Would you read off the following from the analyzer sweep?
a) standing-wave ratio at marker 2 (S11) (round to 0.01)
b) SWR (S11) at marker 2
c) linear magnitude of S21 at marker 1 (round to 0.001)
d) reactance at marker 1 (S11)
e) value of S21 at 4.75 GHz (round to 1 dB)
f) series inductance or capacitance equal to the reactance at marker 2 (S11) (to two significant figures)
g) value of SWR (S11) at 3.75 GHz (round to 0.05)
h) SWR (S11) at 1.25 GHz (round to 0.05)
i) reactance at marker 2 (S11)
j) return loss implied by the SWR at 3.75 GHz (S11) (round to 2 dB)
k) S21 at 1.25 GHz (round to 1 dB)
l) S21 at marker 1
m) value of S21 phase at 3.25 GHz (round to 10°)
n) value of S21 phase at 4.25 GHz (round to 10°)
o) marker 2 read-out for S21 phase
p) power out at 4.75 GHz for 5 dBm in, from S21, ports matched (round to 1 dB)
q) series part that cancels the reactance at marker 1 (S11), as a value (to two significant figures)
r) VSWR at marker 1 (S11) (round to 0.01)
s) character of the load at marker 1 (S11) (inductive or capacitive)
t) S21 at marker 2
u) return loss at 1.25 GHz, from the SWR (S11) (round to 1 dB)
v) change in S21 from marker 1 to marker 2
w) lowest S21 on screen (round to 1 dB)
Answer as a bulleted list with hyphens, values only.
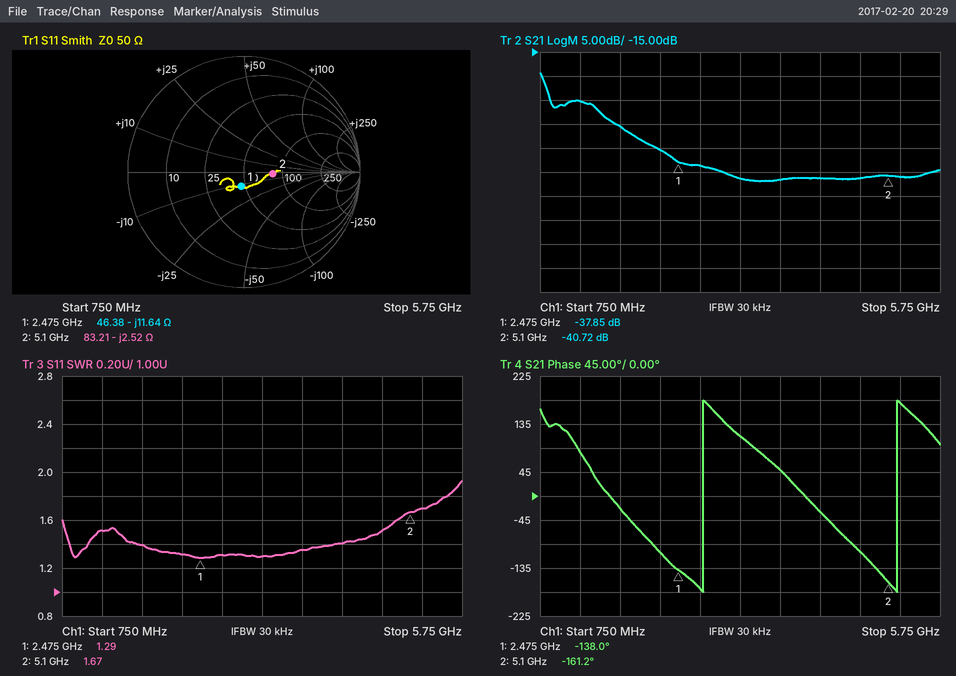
- 1.67
- 1.67
- 0.013
- -11.64 Ω
- -41 dB
- 12 pF
- 1.35
- 1.50
- -2.52 Ω
- 16 dB
- -25 dB
- -37.85 dB
- 110°
- -30°
- -161.2°
- -36 dBm
- 750 pH
- 1.29
- capacitive
- -40.72 dB
- 14 dB
- -2.87 dB
- -42 dB
